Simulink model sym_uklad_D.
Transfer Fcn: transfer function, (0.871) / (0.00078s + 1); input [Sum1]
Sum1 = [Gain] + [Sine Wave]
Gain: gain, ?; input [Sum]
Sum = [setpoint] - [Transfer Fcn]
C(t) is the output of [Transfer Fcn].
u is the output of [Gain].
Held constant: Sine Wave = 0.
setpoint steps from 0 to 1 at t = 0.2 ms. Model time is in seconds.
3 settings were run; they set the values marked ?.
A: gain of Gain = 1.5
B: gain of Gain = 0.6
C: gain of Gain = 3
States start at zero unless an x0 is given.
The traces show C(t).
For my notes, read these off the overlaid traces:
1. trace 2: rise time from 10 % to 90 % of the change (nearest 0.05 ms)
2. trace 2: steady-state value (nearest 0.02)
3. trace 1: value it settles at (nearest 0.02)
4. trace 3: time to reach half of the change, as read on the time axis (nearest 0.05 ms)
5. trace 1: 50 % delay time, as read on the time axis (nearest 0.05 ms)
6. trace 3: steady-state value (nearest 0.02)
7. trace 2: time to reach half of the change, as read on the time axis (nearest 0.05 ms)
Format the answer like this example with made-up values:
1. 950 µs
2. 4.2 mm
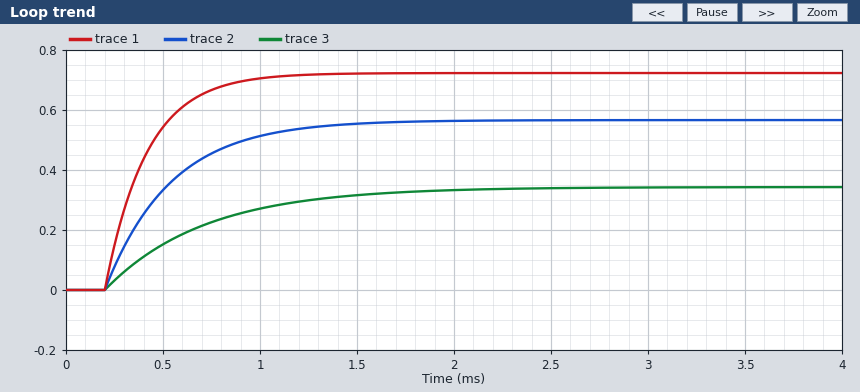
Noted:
1. 0.75 ms
2. 0.56
3. 0.72
4. 0.55 ms
5. 0.35 ms
6. 0.34
7. 0.45 ms
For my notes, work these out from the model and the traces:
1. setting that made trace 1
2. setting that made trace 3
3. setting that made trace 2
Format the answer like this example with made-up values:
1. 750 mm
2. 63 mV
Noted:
1. C
2. B
3. A
